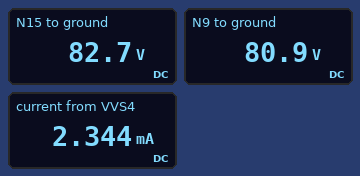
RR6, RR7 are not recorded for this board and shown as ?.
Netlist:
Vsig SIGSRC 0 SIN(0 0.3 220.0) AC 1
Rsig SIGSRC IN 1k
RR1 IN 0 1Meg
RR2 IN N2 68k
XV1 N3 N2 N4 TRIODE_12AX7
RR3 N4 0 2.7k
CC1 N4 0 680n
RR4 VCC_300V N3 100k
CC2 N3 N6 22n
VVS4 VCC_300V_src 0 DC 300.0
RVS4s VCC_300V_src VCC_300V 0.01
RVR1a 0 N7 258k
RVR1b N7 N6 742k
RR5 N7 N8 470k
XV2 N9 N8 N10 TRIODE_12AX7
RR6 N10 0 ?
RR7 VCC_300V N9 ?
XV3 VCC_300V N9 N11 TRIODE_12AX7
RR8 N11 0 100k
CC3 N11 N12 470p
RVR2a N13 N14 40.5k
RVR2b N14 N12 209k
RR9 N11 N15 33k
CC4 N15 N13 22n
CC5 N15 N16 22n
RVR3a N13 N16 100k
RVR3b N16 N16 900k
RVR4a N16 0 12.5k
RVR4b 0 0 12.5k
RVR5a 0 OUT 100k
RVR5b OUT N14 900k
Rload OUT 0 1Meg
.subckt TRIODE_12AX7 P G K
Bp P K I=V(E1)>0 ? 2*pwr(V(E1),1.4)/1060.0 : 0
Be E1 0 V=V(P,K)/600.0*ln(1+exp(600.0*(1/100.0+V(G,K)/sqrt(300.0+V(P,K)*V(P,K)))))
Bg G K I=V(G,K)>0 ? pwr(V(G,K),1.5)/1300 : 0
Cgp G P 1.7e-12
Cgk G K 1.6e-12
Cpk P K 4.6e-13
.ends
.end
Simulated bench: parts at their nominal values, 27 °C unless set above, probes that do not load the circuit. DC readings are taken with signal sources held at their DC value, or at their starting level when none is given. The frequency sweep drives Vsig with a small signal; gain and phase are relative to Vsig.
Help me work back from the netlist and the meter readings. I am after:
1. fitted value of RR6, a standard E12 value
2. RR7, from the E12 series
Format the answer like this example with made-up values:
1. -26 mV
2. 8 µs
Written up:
1. 330 Ω
2. 270 kΩ
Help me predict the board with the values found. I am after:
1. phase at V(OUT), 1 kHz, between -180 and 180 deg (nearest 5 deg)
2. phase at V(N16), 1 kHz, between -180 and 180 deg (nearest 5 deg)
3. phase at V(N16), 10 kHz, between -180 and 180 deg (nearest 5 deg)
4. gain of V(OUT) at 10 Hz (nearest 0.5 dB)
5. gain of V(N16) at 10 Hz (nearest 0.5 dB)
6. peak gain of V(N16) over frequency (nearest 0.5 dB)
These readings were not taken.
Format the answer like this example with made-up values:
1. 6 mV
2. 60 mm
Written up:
1. -30 deg
2. -10 deg
3. -100 deg
4. 13.0 dB
5. 20.5 dB
6. 47.5 dB
